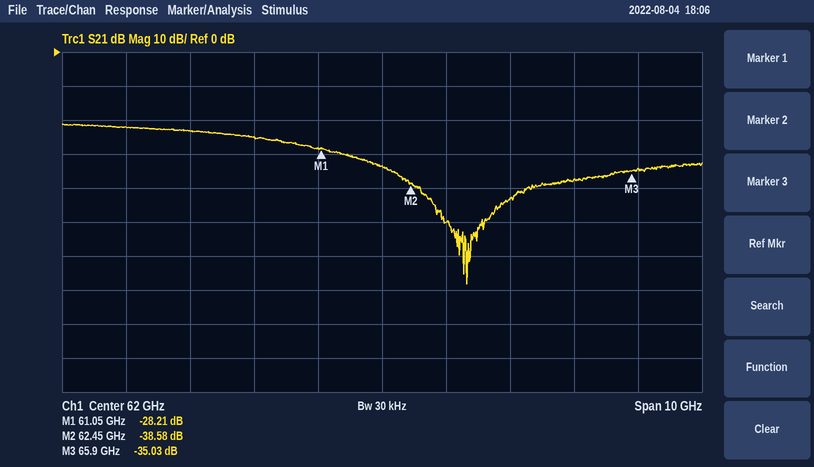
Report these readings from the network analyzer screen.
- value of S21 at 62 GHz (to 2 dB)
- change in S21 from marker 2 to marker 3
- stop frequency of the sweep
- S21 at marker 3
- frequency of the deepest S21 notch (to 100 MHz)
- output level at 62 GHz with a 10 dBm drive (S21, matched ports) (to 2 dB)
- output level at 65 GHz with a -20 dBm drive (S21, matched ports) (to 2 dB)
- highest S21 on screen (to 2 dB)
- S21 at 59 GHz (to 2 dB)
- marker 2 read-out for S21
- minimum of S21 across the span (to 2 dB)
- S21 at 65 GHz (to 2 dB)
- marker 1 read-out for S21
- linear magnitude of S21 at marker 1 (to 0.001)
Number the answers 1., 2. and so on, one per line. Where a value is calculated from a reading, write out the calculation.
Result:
1. -34 dB
2. -35.03 − (-38.58) = 3.55 dB
3. 67 GHz
4. -35.03 dB
5. 63.3 GHz
6. 10 dBm + (-34 dB) = -24 dBm
7. -20 dBm + (-38 dB) = -58 dBm
8. -22 dB
9. -24 dB
10. -38.58 dB
11. -68 dB
12. -38 dB
13. -28.21 dB
14. 10^(-28.21/20) ≈ 0.039
